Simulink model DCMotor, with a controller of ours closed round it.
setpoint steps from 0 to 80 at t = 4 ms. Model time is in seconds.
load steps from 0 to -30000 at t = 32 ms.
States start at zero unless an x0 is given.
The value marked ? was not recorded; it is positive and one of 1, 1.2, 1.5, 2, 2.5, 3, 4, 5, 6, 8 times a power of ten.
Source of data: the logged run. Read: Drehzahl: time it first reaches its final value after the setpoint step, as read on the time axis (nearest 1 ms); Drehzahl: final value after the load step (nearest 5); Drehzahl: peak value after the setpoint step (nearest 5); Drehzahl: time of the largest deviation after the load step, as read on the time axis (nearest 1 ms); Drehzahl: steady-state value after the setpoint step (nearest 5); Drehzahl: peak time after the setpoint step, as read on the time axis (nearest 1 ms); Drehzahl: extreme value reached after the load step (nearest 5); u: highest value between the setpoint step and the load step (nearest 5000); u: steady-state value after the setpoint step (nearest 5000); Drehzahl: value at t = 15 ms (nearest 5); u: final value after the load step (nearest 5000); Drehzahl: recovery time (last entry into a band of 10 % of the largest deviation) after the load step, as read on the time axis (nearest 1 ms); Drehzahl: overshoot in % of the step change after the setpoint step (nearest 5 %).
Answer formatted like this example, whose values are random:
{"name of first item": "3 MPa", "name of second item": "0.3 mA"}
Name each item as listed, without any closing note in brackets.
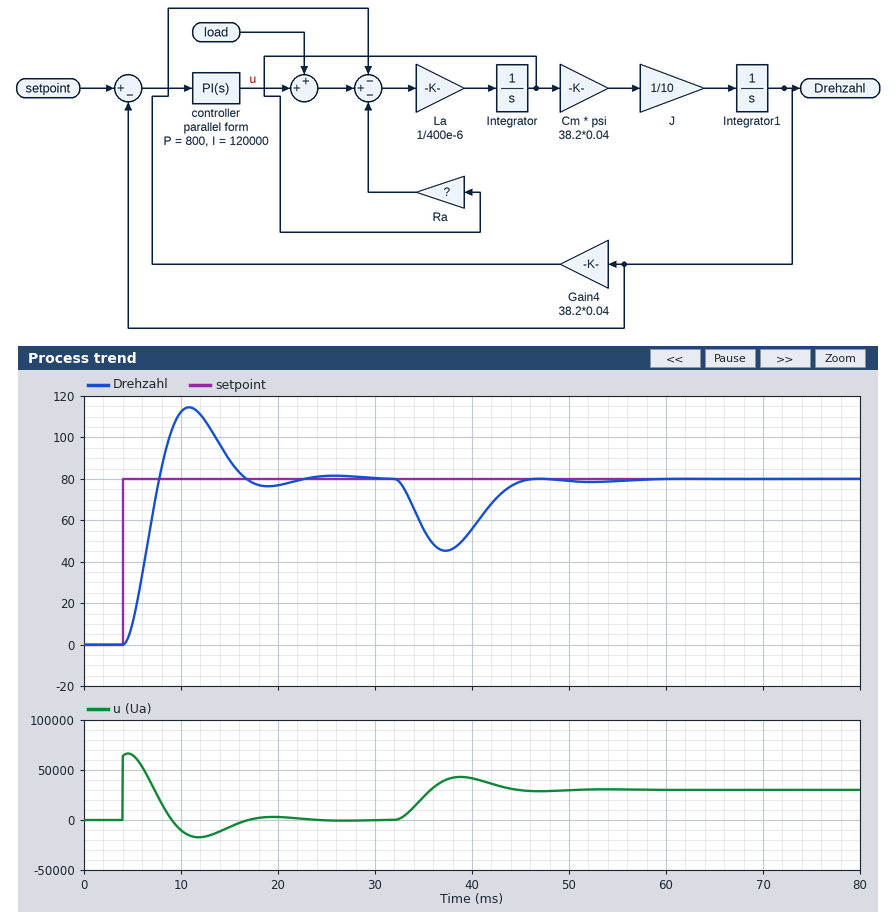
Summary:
{"Drehzahl: time it first reaches its final value after the setpoint step, as read on the time axis": "8 ms", "Drehzahl: final value after the load step": "80", "Drehzahl: peak value after the setpoint step": "115", "Drehzahl: time of the largest deviation after the load step, as read on the time axis": "37 ms", "Drehzahl: steady-state value after the setpoint step": "80", "Drehzahl: peak time after the setpoint step, as read on the time axis": "11 ms", "Drehzahl: extreme value reached after the load step": "45", "u: highest value between the setpoint step and the load step": "65000", "u: steady-state value after the setpoint step": "0", "Drehzahl: value at t = 15 ms": "90", "u: final value after the load step": "30000", "Drehzahl: recovery time (last entry into a band of 10 % of the largest deviation) after the load step, as read on the time axis": "44 ms", "Drehzahl: overshoot in % of the step change after the setpoint step": "45 %"}
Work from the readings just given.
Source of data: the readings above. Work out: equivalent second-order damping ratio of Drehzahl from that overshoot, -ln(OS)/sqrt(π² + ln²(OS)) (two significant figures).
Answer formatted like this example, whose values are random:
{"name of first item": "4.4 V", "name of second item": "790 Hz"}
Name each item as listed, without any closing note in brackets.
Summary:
{"equivalent second-order damping ratio of Drehzahl from that overshoot, -ln(OS)/sqrt(π² + ln²(OS))": "0.25"}
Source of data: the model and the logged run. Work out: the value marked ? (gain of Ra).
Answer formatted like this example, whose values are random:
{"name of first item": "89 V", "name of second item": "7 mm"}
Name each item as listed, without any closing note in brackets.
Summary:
{"the value marked ?": "0.25"}
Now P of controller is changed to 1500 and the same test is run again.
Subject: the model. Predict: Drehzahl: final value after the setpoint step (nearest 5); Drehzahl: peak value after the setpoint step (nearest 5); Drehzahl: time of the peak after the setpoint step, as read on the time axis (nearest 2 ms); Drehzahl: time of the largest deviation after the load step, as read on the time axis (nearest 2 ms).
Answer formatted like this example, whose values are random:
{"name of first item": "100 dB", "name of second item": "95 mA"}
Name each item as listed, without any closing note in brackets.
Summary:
{"Drehzahl: final value after the setpoint step": "80", "Drehzahl: peak value after the setpoint step": "110", "Drehzahl: time of the peak after the setpoint step, as read on the time axis": "8 ms", "Drehzahl: time of the largest deviation after the load step, as read on the time axis": "36 ms"}
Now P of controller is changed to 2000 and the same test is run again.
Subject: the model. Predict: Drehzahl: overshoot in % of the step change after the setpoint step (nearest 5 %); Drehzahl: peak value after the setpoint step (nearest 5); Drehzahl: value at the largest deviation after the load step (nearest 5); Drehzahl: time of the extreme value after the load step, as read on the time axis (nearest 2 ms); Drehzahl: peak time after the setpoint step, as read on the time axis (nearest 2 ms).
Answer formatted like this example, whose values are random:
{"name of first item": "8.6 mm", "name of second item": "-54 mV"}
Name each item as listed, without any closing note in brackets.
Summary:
{"Drehzahl: overshoot in % of the step change after the setpoint step": "40 %", "Drehzahl: peak value after the setpoint step": "110", "Drehzahl: value at the largest deviation after the load step": "60", "Drehzahl: time of the extreme value after the load step, as read on the time axis": "36 ms", "Drehzahl: peak time after the setpoint step, as read on the time axis": "8 ms"}
